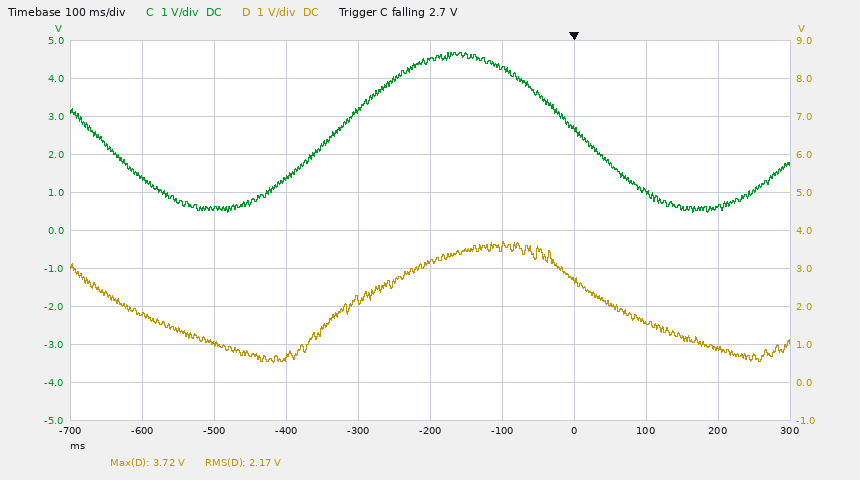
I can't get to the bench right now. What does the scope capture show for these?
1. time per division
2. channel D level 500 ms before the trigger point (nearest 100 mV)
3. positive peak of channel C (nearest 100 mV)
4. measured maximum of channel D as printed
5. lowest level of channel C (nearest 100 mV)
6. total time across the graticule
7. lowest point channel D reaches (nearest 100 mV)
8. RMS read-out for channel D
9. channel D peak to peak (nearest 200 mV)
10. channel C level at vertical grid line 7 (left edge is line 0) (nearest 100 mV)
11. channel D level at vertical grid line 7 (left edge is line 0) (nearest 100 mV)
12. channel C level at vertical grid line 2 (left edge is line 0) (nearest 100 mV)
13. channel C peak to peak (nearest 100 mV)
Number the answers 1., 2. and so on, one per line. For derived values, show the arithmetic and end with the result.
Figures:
1. 100 ms
2. 1.0 V
3. 4.7 V
4. 3.72 V
5. 500 mV
6. 1 s
7. 500 mV
8. 2.17 V
9. 3.2 V
10. 2.7 V
11. 2.7 V
12. 600 mV
13. 4.7 V − (500 mV) = 4.2 V
